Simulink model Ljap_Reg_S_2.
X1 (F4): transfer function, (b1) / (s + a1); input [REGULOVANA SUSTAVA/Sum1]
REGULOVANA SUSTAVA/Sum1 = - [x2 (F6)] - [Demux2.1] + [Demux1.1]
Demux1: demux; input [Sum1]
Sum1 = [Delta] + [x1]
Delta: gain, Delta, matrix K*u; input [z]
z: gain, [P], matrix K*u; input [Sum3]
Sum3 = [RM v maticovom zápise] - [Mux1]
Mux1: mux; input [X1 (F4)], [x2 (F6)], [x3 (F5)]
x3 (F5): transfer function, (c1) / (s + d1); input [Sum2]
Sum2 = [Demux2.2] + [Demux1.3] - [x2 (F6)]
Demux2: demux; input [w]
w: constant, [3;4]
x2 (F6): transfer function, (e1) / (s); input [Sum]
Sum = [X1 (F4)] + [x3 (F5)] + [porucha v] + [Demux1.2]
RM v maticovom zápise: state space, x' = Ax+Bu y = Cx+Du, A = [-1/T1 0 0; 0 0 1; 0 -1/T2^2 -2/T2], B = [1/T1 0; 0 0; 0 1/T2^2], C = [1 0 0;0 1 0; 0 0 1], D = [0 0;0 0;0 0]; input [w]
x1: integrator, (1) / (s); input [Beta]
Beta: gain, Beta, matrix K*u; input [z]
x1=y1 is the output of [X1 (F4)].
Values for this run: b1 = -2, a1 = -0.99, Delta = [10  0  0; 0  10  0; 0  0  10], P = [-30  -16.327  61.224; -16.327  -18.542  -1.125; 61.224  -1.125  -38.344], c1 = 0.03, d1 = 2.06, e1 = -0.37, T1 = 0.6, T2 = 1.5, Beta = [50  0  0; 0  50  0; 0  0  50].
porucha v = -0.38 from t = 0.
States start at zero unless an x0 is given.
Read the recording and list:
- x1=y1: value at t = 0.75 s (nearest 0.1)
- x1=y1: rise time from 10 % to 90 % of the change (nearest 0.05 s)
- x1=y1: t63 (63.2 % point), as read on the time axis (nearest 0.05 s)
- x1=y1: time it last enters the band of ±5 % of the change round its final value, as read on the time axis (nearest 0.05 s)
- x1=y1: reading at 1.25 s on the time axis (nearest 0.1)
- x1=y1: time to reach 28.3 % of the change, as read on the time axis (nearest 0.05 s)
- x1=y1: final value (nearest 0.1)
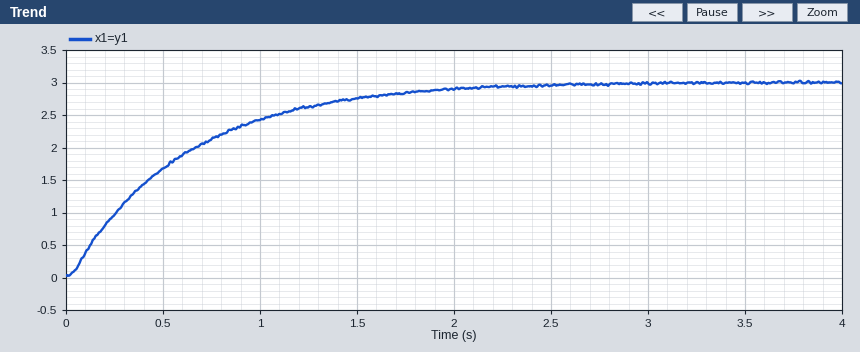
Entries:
2.1
1.30 s
0.60 s
1.80 s
2.6
0.20 s
3.0
